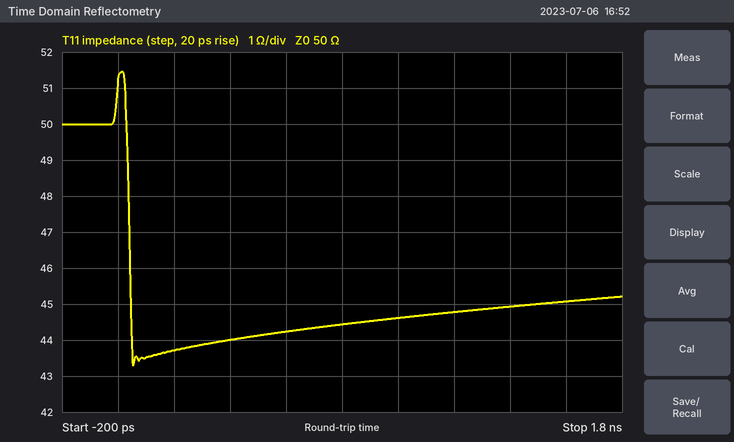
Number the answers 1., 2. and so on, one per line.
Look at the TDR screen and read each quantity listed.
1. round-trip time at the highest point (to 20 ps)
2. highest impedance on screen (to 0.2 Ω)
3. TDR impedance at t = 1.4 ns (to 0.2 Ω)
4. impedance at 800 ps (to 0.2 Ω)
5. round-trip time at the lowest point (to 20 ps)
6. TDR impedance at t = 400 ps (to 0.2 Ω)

1. 20 ps
2. 51.4 Ω
3. 45.0 Ω
4. 44.4 Ω
5. 60 ps
6. 44.0 Ω
